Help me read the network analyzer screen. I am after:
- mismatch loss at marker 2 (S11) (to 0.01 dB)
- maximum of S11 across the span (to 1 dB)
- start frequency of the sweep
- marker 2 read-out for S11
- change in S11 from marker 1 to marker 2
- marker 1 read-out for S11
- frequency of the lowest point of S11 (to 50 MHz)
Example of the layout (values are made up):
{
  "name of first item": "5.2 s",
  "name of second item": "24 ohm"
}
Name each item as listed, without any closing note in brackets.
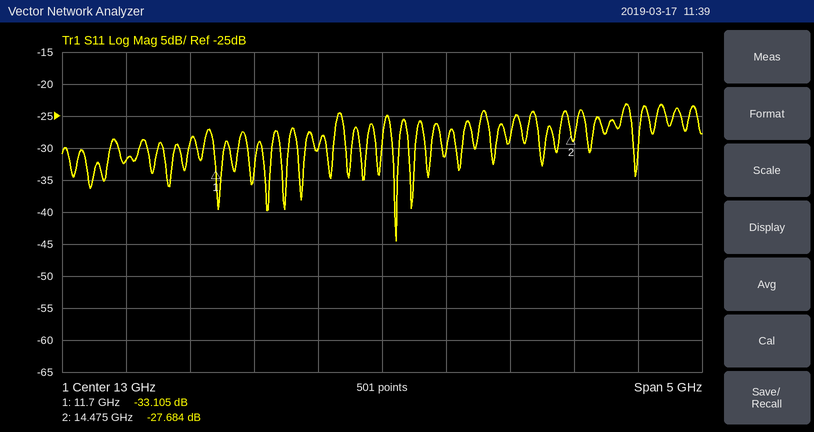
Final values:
{
  "mismatch loss at marker 2 (S11)": "0.01 dB",
  "maximum of S11 across the span": "-23 dB",
  "start frequency of the sweep": "10.5 GHz",
  "marker 2 read-out for S11": "-27.684 dB",
  "change in S11 from marker 1 to marker 2": "5.421 dB",
  "marker 1 read-out for S11": "-33.105 dB",
  "frequency of the lowest point of S11": "13.10 GHz"
}
